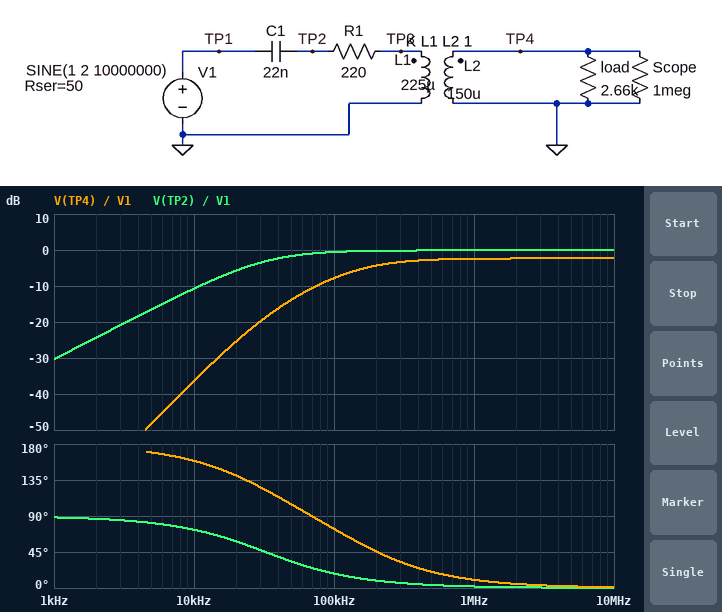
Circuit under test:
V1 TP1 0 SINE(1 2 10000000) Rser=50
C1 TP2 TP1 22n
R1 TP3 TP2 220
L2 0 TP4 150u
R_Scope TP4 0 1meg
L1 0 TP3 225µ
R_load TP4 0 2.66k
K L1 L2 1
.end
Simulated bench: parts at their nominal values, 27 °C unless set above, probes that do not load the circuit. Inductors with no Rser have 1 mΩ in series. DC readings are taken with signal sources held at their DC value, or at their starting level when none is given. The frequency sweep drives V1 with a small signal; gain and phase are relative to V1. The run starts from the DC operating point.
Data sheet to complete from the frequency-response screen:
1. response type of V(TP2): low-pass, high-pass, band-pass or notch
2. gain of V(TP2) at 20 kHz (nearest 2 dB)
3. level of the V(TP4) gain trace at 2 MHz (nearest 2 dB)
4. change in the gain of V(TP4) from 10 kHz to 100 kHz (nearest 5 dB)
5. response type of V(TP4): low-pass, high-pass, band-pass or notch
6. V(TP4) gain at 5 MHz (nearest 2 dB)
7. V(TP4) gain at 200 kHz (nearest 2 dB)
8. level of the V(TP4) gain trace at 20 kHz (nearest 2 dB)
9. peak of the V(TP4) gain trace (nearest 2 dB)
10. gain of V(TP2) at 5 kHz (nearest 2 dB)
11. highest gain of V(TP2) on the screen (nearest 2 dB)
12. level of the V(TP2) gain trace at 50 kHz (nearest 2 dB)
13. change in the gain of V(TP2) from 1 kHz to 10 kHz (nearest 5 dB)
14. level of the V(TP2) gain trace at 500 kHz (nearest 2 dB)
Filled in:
high-pass
-6 dB
-2 dB
30 dB
high-pass
-2 dB
-4 dB
-26 dB
-2 dB
-16 dB
0 dB
-2 dB
20 dB
0 dB
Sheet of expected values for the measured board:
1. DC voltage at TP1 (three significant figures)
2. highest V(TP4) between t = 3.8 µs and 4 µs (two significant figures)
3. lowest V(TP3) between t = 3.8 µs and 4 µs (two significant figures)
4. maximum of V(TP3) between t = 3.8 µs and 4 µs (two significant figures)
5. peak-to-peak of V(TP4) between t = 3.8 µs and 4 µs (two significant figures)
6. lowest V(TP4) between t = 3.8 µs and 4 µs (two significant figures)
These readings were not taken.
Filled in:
1.00 V
1.5 V
-1.9 V
1.9 V
3.1 V
-1.5 V
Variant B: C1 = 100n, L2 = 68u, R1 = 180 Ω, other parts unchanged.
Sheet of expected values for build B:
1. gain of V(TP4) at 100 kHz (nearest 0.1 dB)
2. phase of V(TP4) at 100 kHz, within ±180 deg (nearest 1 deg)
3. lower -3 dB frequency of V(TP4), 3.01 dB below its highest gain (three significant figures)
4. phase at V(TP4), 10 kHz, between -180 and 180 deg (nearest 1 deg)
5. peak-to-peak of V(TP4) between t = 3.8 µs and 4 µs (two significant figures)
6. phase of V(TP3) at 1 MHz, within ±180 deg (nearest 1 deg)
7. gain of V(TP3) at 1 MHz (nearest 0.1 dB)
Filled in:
-10.6 dB
61 deg
152 kHz
122 deg
2.1 V
9 deg
-0.3 dB
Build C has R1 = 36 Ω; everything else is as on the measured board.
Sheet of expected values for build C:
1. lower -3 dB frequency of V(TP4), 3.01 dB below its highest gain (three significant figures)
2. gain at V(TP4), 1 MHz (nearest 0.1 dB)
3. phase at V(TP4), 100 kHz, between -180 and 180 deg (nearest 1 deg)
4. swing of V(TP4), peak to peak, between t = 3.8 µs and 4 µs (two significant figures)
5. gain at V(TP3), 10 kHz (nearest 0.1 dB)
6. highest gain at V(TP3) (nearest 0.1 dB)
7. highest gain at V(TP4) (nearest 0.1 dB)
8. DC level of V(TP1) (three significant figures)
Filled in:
59.7 kHz
-1.9 dB
51 deg
3.2 V
-34.1 dB
2.0 dB
0.2 dB
1.00 V
